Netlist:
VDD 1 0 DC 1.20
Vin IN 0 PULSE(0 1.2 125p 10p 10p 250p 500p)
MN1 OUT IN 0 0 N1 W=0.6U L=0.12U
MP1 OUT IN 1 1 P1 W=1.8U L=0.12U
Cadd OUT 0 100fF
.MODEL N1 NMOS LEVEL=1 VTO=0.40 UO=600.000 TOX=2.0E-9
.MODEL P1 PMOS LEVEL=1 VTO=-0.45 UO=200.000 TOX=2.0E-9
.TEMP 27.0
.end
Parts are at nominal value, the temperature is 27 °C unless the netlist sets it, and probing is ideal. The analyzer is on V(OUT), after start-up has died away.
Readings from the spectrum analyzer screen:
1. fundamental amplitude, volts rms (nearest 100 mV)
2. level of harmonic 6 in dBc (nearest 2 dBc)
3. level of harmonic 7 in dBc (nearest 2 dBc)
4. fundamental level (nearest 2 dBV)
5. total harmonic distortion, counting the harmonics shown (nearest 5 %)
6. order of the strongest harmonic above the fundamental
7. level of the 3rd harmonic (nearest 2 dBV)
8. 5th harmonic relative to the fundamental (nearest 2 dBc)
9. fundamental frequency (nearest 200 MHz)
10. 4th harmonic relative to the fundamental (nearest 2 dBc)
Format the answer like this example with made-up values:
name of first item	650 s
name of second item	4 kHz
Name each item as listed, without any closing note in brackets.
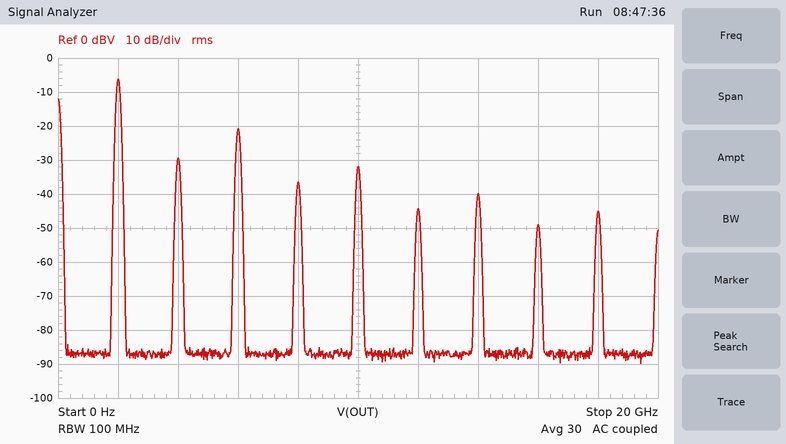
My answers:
fundamental amplitude, volts rms	500 mV
level of harmonic 6 in dBc	-38 dBc
level of harmonic 7 in dBc	-34 dBc
fundamental level	-6 dBV
total harmonic distortion, counting the harmonics shown	20 %
order of the strongest harmonic above the fundamental	3
level of the 3rd harmonic	-20 dBV
5th harmonic relative to the fundamental	-26 dBc
fundamental frequency	2.0 GHz
4th harmonic relative to the fundamental	-30 dBc
